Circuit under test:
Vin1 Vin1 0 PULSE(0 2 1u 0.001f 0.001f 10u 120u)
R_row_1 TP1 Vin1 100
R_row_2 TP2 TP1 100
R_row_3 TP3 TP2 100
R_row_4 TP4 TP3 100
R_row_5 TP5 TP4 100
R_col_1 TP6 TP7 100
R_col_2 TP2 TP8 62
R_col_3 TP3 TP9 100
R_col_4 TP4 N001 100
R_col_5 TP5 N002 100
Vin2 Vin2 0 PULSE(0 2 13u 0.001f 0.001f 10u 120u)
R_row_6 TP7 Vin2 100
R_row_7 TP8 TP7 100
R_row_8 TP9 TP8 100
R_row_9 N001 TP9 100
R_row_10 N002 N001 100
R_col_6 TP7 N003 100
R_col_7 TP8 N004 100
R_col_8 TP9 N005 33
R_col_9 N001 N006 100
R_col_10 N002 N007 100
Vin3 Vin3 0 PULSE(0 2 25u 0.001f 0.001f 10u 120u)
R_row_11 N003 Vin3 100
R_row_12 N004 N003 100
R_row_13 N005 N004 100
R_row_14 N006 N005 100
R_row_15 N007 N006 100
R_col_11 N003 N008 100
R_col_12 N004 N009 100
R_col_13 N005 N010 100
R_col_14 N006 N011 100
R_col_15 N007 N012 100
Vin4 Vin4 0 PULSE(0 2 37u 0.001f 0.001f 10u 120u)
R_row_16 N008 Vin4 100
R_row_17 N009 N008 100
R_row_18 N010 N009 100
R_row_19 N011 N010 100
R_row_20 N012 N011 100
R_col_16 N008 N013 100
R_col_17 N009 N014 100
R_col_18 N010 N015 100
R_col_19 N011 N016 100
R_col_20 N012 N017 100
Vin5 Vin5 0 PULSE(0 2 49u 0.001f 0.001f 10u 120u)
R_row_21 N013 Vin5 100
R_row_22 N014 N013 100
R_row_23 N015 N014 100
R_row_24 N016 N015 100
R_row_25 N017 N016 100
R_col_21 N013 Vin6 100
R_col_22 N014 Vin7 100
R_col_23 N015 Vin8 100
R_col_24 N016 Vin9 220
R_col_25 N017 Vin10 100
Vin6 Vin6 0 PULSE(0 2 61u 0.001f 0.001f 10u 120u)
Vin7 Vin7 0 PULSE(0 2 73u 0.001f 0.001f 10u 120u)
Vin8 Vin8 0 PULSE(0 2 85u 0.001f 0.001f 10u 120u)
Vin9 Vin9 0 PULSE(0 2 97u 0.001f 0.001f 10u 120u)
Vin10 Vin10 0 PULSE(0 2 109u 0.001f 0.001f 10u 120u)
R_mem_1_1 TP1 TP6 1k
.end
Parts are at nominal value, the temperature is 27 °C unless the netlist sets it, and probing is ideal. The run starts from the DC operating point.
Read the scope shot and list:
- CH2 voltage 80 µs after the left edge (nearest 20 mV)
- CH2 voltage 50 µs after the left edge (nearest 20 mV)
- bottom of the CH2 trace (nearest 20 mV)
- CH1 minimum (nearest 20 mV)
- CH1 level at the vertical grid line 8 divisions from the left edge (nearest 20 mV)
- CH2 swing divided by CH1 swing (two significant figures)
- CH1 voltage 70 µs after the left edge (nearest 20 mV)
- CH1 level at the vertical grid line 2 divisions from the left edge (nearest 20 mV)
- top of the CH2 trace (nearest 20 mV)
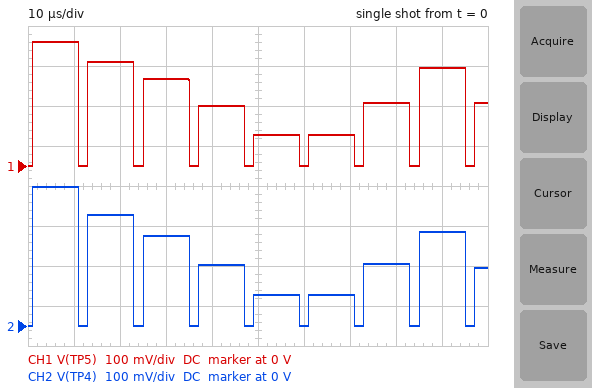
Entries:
160 mV
80 mV
0 V
0 V
160 mV
1.1
80 mV
260 mV
340 mV
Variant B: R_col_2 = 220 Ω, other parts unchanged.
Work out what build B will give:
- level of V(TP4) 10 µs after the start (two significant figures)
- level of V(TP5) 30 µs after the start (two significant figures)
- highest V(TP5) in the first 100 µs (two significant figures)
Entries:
380 mV
210 mV
330 mV
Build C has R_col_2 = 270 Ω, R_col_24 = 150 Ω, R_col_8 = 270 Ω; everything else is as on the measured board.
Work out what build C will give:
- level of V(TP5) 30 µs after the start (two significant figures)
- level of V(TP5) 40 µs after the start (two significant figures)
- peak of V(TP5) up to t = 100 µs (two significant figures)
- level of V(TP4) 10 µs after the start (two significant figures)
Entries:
210 mV
140 mV
360 mV
410 mV
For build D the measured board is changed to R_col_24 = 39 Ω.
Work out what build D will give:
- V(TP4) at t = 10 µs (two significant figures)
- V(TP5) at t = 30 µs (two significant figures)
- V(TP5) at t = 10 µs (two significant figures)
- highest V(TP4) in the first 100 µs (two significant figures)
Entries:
330 mV
200 mV
290 mV
400 mV
